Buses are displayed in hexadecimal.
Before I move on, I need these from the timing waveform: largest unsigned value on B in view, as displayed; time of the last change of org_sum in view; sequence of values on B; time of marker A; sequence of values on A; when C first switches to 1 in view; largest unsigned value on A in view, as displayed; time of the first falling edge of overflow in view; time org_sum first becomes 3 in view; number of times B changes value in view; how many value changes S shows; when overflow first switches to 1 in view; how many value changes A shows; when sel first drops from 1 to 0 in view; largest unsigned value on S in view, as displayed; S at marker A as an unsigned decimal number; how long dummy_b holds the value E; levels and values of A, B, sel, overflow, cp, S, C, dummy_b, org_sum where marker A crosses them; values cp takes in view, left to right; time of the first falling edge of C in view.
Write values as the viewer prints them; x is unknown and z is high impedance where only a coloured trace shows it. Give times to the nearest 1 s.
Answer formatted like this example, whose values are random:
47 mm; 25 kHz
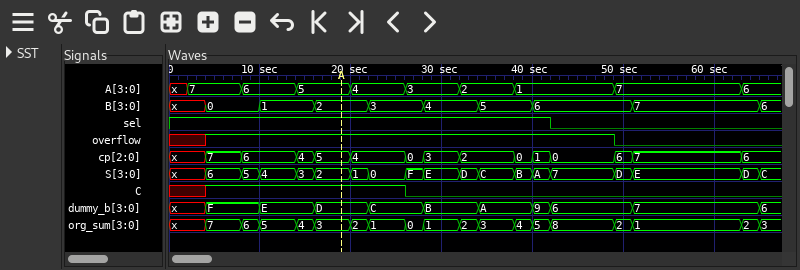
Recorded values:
7; 65 s; x, 0, 1, 2, 3, 4, 5, 6, 7, 6; 19 s; x, 7, 6, 5, 4, 3, 2, 1, 7, 6; 4 s; 7; 49 s; 16 s; 9; 18; 4 s; 9; 42 s; F; 2; 6 s; A=5, B=2, sel=1, overflow=1, cp=5, S=2, C=1, dummy_b=D, org_sum=3; x, 7, 6, 4, 5, 4, 0, 3, 2, 0, 1, 0, 6, 7, 6; 26 s
